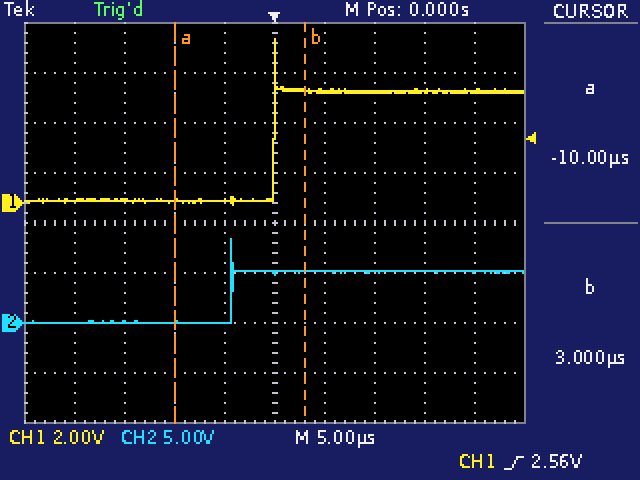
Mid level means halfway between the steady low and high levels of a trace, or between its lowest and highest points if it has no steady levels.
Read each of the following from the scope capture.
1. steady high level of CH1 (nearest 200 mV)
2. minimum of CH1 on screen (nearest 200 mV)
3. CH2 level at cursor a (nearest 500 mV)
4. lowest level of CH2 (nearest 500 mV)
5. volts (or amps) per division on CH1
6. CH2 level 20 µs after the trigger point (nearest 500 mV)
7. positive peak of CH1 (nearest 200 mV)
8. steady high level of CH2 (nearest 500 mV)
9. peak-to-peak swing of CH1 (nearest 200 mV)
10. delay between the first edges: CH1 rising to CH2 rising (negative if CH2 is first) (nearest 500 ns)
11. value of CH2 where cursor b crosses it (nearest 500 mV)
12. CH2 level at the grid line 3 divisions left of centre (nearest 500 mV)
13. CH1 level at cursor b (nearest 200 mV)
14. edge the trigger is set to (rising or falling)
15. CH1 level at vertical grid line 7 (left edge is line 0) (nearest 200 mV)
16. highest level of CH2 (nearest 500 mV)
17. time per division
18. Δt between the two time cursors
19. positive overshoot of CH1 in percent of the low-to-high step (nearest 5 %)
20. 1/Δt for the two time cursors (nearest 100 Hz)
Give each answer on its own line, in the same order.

4.4 V
0.0 V
0.0 V
0.0 V
2 V
5.0 V
6.6 V
5.0 V
6.6 V
-4.5 µs
5.0 V
0.0 V
4.4 V
rising
4.4 V
8.5 V
5 µs
13.0 µs
50 %
76.9 kHz
